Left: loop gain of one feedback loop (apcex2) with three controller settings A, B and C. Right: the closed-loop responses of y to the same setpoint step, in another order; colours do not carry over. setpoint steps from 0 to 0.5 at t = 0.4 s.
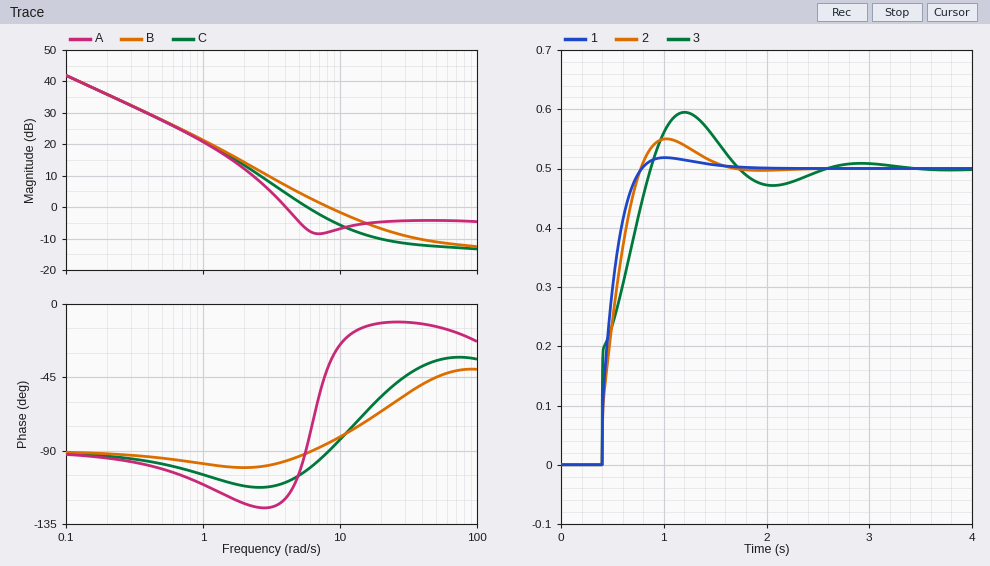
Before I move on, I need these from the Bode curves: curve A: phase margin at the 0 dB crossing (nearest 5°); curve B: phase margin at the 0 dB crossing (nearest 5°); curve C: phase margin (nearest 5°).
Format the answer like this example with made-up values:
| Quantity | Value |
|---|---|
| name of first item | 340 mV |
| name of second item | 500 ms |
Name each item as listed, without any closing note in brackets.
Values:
| Quantity | Value |
|---|---|
| curve A: phase margin at the 0 dB crossing | 60° |
| curve B: phase margin at the 0 dB crossing | 95° |
| curve C: phase margin | 80° |
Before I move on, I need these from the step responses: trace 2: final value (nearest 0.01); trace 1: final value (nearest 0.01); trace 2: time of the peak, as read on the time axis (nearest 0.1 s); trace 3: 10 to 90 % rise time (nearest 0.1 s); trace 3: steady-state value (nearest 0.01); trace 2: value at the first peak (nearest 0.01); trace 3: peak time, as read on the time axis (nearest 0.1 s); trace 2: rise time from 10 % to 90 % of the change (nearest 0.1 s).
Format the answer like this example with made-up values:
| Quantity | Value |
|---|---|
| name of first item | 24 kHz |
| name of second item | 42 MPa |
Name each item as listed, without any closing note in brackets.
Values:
| Quantity | Value |
|---|---|
| trace 2: final value | 0.50 |
| trace 1: final value | 0.50 |
| trace 2: time of the peak, as read on the time axis | 1.0 s |
| trace 3: 10 to 90 % rise time | 0.4 s |
| trace 3: steady-state value | 0.50 |
| trace 2: value at the first peak | 0.55 |
| trace 3: peak time, as read on the time axis | 1.2 s |
| trace 2: rise time from 10 % to 90 % of the change | 0.3 s |
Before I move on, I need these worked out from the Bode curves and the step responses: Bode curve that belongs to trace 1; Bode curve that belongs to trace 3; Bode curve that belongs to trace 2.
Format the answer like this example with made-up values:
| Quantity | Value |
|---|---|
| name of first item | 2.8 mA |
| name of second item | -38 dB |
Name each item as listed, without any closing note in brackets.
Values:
| Quantity | Value |
|---|---|
| Bode curve that belongs to trace 1 | B |
| Bode curve that belongs to trace 3 | A |
| Bode curve that belongs to trace 2 | C |
